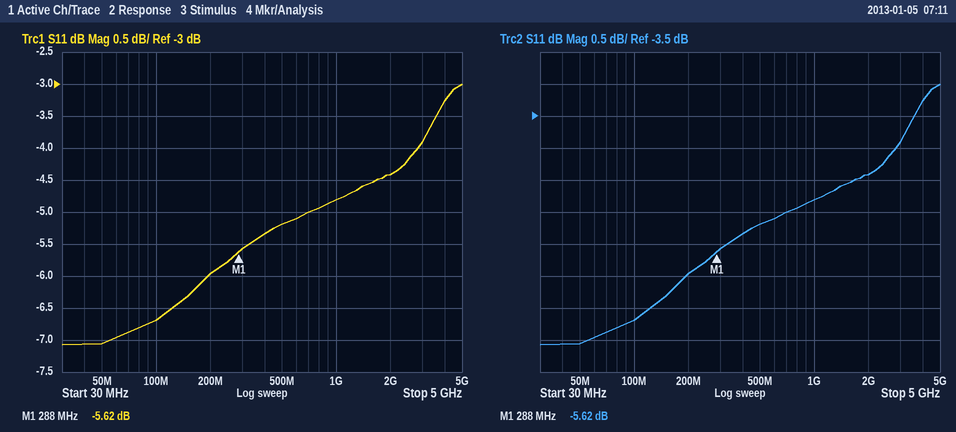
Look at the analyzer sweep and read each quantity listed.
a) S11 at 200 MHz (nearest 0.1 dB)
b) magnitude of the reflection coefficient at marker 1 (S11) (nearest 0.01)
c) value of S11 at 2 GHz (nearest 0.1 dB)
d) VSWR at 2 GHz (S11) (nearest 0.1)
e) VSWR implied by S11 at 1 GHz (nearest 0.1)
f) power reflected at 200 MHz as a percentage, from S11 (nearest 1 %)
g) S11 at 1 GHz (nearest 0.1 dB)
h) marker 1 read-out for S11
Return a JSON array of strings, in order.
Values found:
["-6.0 dB", "0.52", "-4.4 dB", "4.0", "3.7", "25 %", "-4.8 dB", "-5.62 dB"]
